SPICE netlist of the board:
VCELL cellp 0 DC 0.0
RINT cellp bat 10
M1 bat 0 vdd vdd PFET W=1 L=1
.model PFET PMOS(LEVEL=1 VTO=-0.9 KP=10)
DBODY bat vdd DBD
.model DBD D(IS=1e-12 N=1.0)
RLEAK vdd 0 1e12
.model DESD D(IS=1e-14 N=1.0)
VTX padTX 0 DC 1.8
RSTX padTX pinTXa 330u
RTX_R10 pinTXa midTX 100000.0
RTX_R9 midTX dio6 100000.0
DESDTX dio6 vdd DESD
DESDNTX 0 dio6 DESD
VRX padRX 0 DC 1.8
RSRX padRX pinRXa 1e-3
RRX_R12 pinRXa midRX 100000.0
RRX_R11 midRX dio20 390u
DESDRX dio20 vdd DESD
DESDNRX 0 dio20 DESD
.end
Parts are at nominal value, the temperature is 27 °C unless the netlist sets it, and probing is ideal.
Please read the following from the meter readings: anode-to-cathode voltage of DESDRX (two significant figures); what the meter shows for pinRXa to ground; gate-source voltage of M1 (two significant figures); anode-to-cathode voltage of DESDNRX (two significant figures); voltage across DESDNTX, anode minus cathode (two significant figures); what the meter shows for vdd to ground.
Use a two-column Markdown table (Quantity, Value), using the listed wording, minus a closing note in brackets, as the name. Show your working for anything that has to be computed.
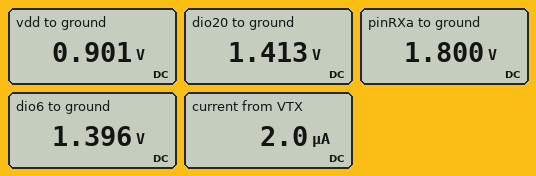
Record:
| Quantity | Value |
|---|---|
| anode-to-cathode voltage of DESDRX | 1.413 V - 901 mV = 510 mV |
| what the meter shows for pinRXa to ground | 1.800 V |
| gate-source voltage of M1 | 0 V - 901 mV = -900 mV |
| anode-to-cathode voltage of DESDNRX | 0 V - 1.413 V = -1.4 V |
| voltage across DESDNTX, anode minus cathode | 0 V - 1.396 V = -1.4 V |
| what the meter shows for vdd to ground | 0.901 V |
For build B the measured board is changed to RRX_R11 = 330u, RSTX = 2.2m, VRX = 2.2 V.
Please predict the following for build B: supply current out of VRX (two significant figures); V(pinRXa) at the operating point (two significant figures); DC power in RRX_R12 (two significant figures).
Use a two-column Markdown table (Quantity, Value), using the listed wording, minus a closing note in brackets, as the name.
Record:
| Quantity | Value |
|---|---|
| supply current out of VRX | 7.7 µA |
| V(pinRXa) at the operating point | 2.2 V |
| DC power in RRX_R12 | 5.9 µW |
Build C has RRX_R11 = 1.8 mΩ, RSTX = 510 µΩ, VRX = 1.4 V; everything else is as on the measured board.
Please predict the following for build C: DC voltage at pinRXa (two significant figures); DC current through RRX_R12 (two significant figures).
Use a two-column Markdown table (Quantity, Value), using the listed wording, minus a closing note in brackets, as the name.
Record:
| Quantity | Value |
|---|---|
| DC voltage at pinRXa | 1.4 V |
| DC current through RRX_R12 | 440 nA |
